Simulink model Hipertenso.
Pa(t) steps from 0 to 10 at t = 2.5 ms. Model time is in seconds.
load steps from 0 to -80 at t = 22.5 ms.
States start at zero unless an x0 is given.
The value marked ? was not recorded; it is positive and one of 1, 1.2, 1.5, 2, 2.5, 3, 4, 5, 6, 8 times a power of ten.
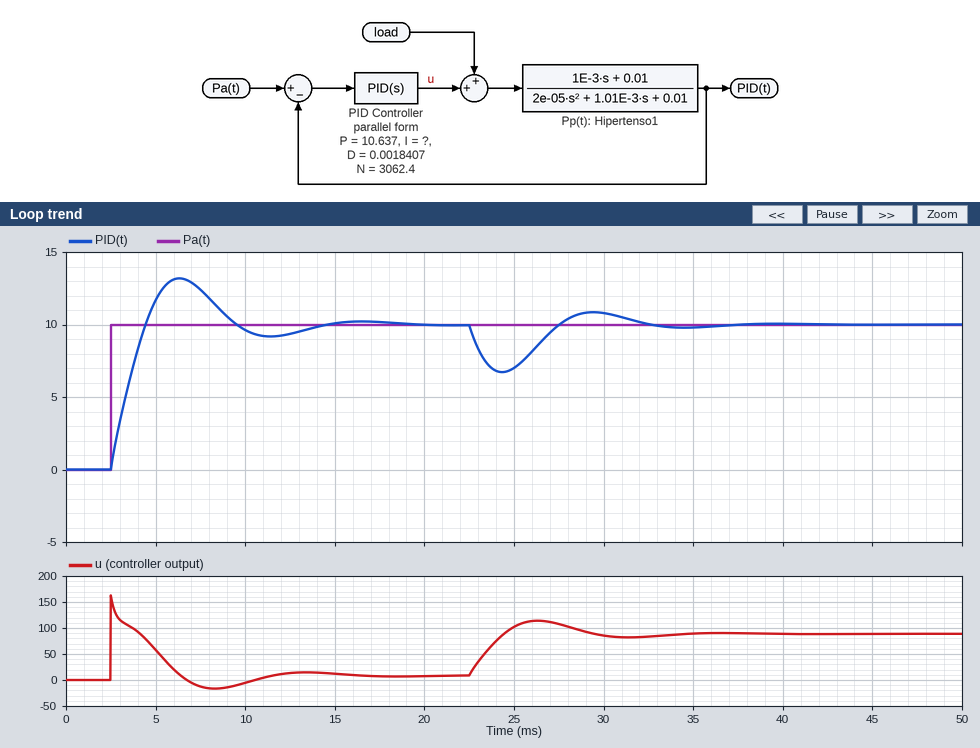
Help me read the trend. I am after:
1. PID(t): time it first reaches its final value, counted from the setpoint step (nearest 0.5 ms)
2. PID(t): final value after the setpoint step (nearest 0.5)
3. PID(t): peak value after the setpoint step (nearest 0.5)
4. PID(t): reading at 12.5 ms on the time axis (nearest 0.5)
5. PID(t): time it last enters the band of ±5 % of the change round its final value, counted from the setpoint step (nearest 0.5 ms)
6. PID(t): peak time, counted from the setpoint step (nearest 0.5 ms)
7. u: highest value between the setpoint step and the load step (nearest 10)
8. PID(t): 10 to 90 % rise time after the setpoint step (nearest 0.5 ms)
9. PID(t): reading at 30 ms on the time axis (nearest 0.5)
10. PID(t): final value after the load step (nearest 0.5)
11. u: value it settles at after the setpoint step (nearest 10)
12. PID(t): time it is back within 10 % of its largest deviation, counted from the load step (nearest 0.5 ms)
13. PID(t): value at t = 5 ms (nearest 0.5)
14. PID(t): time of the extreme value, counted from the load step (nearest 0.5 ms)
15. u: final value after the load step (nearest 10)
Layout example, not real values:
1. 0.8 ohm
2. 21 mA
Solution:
1. 2.0 ms
2. 10.0
3. 13.0
4. 9.5
5. 10.5 ms
6. 4.0 ms
7. 160
8. 1.5 ms
9. 11.0
10. 10.0
11. 10
12. 9.0 ms
13. 11.5
14. 2.0 ms
15. 90
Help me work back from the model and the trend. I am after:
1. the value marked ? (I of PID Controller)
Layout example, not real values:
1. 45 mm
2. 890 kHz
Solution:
1. 10000
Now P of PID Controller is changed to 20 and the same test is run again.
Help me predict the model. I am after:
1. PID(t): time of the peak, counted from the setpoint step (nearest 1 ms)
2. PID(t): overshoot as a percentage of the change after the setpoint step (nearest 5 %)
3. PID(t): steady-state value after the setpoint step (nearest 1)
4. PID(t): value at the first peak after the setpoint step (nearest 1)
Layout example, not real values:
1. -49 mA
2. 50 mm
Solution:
1. 3 ms
2. 15 %
3. 10
4. 12
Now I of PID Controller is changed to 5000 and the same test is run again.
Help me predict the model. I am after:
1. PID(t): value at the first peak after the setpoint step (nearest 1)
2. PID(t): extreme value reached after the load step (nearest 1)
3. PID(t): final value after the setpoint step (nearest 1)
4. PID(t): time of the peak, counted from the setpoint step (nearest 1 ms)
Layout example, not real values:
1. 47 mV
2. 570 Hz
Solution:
1. 12
2. 6
3. 10
4. 5 ms
